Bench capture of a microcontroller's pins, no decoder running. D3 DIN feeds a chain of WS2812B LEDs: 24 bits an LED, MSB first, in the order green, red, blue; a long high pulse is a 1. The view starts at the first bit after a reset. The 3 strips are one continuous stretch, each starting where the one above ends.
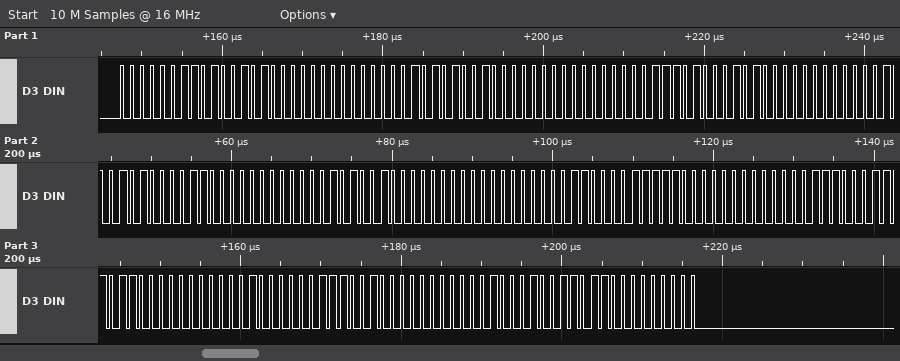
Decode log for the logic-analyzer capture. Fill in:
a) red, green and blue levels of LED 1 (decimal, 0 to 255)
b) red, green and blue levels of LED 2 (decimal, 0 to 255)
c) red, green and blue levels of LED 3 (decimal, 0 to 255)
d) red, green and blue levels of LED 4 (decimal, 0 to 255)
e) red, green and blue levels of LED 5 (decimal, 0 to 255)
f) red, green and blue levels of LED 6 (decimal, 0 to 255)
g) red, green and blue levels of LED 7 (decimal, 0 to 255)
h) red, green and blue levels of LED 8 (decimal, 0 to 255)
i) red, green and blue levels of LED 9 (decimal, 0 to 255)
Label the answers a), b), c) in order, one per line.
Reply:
a) 74, 3, 0
b) 72, 5, 0
c) 69, 7, 0
d) 67, 9, 0
e) 64, 10, 0
f) 62, 12, 0
g) 59, 14, 0
h) 57, 16, 0
i) 54, 17, 0
